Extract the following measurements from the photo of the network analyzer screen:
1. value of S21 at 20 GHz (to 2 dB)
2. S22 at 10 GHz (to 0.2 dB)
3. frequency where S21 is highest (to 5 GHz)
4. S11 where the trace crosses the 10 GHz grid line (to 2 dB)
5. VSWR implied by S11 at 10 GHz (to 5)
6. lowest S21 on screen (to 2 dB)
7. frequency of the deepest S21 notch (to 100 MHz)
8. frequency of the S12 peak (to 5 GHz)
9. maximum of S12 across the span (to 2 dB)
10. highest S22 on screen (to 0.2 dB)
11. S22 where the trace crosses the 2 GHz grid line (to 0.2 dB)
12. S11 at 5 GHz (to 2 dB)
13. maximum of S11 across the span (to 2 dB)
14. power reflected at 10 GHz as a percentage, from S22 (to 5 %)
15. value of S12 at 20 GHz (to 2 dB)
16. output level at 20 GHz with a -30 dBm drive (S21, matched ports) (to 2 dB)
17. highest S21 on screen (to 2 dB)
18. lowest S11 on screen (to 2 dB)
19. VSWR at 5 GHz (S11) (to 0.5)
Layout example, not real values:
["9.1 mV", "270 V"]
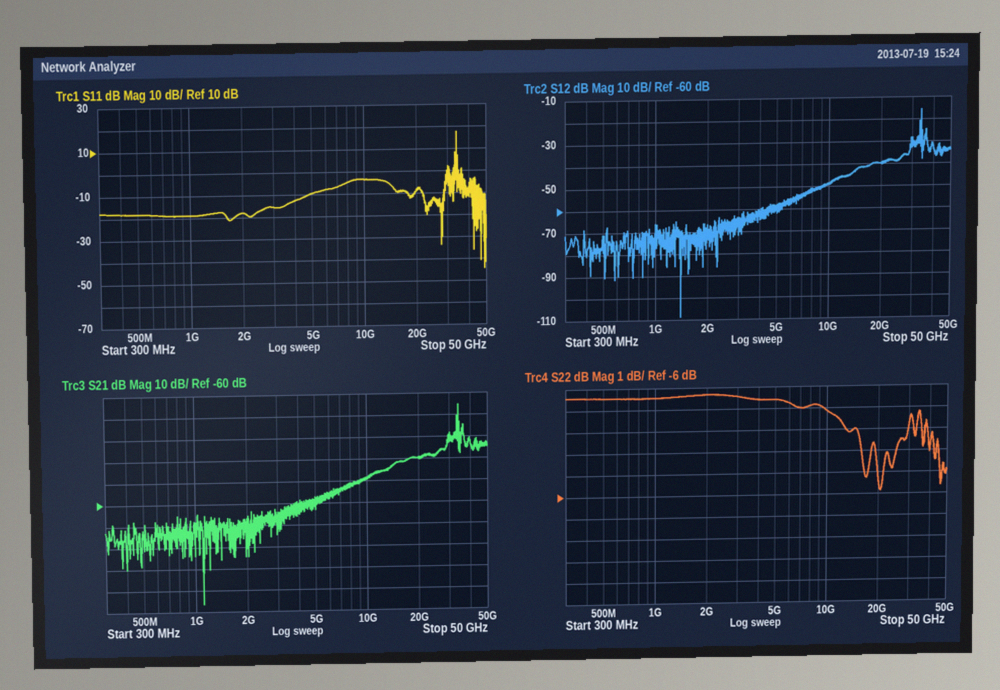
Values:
["-40 dB", "-2.2 dB", "35 GHz", "-4 dB", "5", "-106 dB", "1.1 GHz", "35 GHz", "-16 dB", "-1.4 dB", "-1.4 dB", "-10 dB", "18 dB", "60 %", "-40 dB", "-70 dBm", "-16 dB", "-44 dB", "2.0"]
